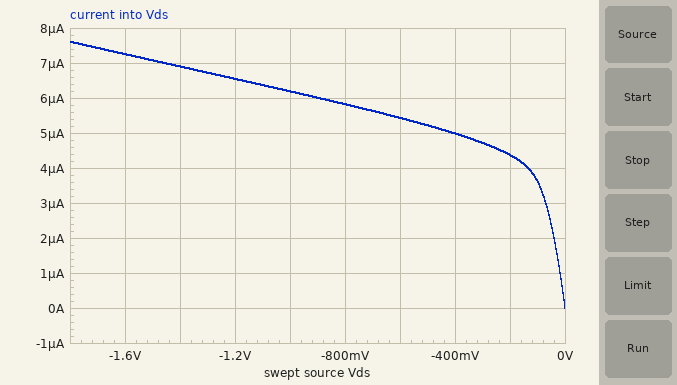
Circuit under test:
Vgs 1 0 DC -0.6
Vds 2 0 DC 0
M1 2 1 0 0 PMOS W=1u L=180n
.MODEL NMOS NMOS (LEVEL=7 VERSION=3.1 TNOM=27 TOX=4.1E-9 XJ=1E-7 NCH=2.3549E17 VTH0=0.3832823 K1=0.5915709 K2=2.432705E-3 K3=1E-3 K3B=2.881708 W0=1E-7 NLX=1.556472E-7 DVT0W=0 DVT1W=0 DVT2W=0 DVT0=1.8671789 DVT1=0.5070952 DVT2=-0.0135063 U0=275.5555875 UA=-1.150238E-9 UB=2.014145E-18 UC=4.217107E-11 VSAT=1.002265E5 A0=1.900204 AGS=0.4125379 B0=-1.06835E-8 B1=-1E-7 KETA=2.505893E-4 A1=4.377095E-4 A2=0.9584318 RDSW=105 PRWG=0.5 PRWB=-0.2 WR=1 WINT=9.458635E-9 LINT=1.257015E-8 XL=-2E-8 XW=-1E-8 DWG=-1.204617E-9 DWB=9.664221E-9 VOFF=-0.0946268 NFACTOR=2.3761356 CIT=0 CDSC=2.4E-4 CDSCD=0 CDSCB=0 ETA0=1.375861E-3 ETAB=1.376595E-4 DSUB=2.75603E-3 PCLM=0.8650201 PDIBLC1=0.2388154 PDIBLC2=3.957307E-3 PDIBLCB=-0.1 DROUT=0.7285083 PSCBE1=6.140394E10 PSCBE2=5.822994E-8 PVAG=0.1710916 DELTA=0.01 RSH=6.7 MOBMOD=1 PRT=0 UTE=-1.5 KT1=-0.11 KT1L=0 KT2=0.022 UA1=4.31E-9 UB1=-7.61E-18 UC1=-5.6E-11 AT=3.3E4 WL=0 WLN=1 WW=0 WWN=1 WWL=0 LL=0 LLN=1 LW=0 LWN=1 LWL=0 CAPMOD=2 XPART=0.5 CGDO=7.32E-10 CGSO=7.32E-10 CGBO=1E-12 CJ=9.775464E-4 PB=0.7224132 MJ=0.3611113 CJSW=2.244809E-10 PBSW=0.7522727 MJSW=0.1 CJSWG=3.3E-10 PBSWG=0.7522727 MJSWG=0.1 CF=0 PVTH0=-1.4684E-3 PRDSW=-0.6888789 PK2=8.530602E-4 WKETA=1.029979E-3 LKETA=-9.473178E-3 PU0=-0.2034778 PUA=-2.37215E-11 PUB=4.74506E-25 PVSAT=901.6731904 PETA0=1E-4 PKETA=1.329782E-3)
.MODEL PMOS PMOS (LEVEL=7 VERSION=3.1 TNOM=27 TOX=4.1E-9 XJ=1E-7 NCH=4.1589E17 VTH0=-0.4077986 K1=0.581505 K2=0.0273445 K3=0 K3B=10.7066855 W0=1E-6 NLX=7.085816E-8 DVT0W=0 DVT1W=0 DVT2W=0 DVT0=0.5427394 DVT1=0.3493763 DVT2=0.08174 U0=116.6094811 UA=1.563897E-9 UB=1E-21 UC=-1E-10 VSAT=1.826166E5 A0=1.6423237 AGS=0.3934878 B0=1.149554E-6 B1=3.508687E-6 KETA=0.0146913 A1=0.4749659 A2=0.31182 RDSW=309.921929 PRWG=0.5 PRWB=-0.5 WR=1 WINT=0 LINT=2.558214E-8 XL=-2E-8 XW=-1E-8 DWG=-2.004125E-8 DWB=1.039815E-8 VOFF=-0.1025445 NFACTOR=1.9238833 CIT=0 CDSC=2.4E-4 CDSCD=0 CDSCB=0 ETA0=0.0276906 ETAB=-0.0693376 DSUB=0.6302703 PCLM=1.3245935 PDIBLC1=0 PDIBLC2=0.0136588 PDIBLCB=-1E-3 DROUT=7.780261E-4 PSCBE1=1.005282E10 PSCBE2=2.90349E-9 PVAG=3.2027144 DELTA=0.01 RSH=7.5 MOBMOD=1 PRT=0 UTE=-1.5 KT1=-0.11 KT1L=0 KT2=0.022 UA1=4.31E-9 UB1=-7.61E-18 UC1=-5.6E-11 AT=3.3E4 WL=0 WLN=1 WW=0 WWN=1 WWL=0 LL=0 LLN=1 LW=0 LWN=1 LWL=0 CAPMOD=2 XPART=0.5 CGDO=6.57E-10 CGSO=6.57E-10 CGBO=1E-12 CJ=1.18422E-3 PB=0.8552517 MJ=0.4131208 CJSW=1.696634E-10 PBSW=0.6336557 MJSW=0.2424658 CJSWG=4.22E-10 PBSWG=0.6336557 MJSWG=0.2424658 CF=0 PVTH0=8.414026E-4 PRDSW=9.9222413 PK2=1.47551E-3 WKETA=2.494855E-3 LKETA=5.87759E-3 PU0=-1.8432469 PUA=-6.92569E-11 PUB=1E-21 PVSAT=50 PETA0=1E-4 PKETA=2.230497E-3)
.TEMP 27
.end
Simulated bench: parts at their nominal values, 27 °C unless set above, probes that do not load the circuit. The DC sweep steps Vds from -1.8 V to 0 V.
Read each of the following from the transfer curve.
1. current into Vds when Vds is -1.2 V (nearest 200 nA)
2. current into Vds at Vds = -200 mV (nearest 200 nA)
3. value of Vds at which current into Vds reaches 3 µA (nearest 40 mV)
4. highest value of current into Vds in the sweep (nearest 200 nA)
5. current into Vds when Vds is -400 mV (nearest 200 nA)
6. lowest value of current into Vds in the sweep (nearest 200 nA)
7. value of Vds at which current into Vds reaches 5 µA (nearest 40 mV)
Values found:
6.6 µA
4.4 µA
-80 mV
7.6 µA
5.0 µA
0 A
-400 mV
